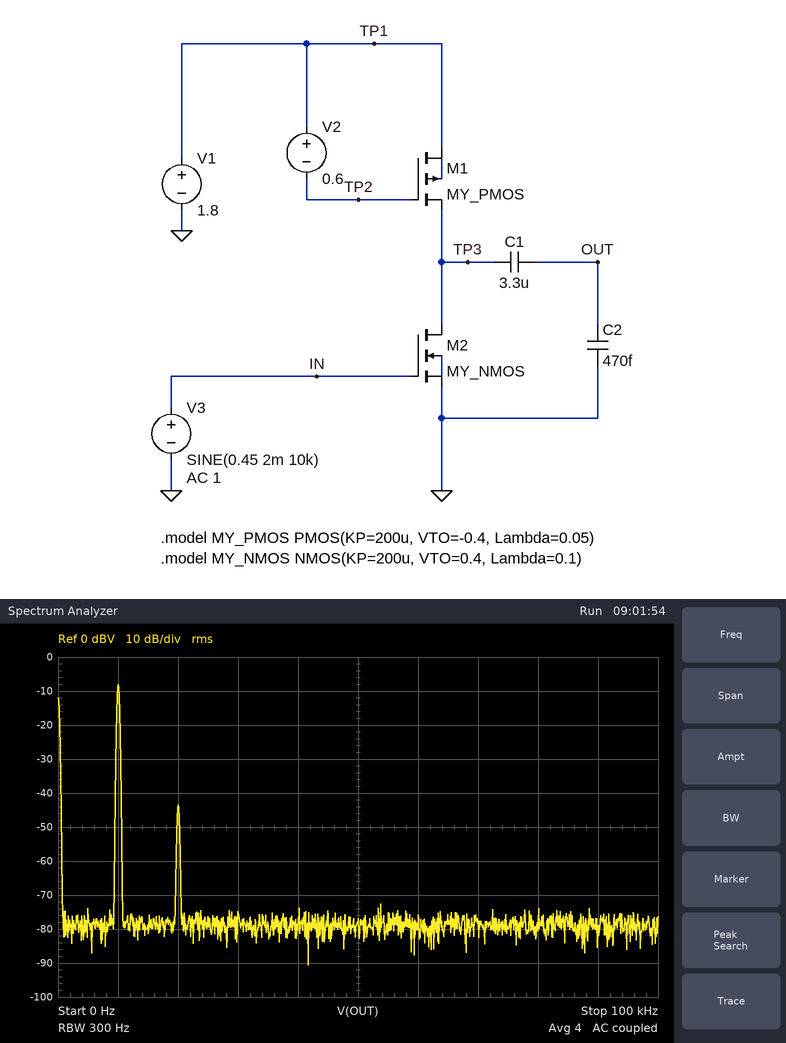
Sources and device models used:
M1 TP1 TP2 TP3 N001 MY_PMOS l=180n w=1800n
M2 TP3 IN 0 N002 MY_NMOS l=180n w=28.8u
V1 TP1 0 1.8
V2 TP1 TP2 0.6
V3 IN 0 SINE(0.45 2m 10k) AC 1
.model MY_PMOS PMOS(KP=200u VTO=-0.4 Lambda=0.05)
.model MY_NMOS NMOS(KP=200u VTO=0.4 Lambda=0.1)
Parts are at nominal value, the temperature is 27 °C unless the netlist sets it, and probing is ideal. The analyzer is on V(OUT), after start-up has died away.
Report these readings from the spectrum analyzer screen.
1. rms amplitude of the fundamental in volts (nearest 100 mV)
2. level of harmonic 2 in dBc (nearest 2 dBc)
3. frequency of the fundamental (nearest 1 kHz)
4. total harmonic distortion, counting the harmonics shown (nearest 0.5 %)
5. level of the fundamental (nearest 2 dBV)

400 mV
-36 dBc
10 kHz
1.5 %
-8 dBV
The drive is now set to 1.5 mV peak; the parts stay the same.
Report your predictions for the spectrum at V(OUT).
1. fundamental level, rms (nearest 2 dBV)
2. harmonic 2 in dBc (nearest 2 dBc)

-10 dBV
-38 dBc
